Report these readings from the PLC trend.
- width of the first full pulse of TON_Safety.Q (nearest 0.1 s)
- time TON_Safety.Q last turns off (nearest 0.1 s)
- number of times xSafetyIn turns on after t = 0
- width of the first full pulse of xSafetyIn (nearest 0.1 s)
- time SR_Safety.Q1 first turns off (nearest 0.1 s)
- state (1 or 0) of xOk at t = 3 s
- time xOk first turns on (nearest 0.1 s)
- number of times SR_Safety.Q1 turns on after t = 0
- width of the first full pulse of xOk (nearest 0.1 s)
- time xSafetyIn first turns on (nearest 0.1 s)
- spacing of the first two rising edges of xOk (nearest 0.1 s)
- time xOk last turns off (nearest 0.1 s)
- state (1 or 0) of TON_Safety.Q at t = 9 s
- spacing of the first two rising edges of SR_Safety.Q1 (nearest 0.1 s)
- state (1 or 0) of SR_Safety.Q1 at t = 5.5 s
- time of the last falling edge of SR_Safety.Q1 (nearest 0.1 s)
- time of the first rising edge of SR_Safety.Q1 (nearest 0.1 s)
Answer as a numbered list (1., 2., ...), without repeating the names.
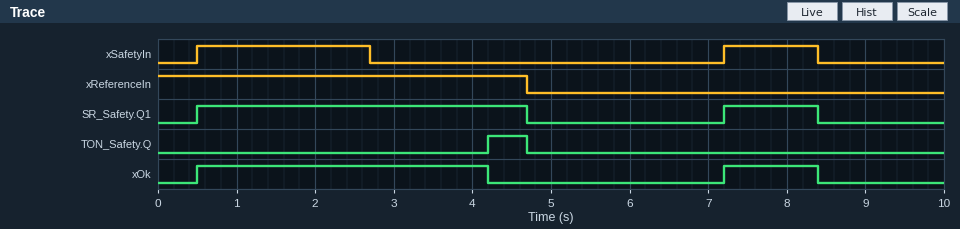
1. 0.5 s
2. 4.7 s
3. 2
4. 2.2 s
5. 4.7 s
6. 1
7. 0.5 s
8. 2
9. 3.7 s
10. 0.5 s
11. 6.7 s
12. 8.4 s
13. 0
14. 6.7 s
15. 0
16. 8.4 s
17. 0.5 s
